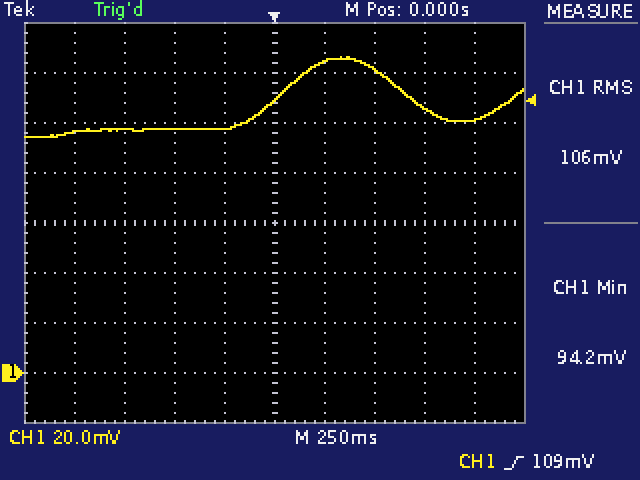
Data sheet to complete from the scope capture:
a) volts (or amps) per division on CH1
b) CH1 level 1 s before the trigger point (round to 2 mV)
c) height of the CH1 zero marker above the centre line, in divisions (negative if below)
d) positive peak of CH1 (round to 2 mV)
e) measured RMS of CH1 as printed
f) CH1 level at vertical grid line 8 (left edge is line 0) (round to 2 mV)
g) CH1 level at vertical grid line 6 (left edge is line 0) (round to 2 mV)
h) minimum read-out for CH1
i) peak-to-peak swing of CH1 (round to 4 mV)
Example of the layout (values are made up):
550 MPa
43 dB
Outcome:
20 mV
96 mV
-3.0 div
126 mV
106 mV
106 mV
124 mV
94.2 mV
32 mV
